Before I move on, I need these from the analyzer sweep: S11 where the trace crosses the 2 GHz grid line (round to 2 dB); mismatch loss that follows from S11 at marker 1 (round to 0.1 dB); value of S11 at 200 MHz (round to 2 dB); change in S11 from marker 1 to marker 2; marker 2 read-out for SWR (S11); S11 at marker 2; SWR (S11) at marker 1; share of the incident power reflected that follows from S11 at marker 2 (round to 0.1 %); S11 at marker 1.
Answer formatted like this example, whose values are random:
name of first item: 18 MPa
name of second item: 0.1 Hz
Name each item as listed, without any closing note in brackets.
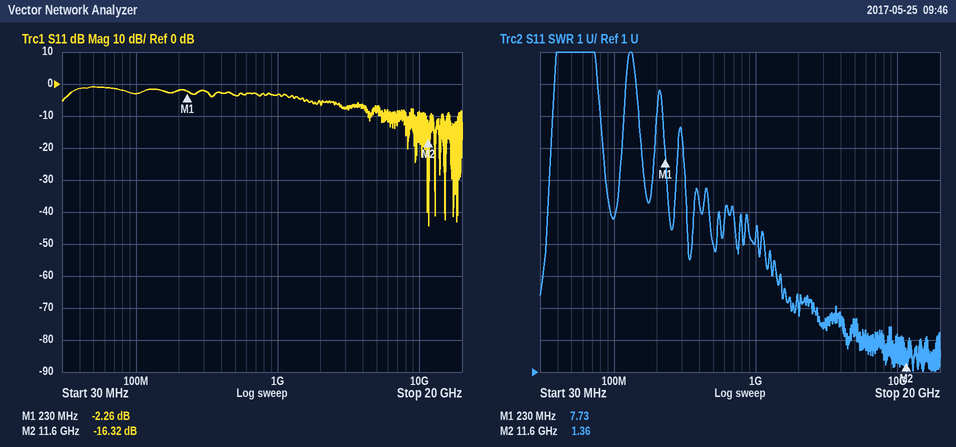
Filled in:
S11 where the trace crosses the 2 GHz grid line: -6 dB
mismatch loss that follows from S11 at marker 1: 3.9 dB
value of S11 at 200 MHz: -2 dB
change in S11 from marker 1 to marker 2: -14.06 dB
marker 2 read-out for SWR: 1.36
S11 at marker 2: -16.32 dB
SWR (S11) at marker 1: 7.73
share of the incident power reflected that follows from S11 at marker 2: 2.3 %
S11 at marker 1: -2.26 dB
